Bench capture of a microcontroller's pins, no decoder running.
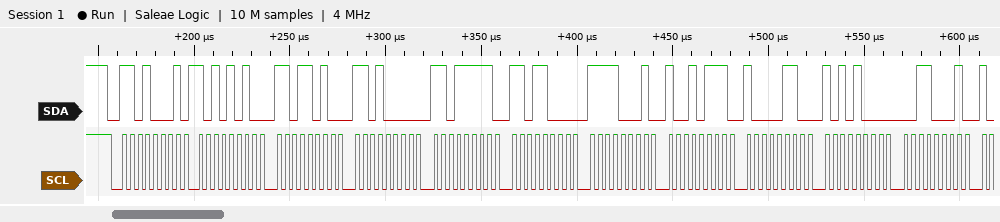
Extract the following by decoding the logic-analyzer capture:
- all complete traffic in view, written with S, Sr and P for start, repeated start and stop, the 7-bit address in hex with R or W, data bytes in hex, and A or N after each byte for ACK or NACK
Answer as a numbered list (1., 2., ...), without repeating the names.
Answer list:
1. S 68R A AA A DA A D0 A DF A D8 A F1 A 97 A 86 A A8 A 31 A
